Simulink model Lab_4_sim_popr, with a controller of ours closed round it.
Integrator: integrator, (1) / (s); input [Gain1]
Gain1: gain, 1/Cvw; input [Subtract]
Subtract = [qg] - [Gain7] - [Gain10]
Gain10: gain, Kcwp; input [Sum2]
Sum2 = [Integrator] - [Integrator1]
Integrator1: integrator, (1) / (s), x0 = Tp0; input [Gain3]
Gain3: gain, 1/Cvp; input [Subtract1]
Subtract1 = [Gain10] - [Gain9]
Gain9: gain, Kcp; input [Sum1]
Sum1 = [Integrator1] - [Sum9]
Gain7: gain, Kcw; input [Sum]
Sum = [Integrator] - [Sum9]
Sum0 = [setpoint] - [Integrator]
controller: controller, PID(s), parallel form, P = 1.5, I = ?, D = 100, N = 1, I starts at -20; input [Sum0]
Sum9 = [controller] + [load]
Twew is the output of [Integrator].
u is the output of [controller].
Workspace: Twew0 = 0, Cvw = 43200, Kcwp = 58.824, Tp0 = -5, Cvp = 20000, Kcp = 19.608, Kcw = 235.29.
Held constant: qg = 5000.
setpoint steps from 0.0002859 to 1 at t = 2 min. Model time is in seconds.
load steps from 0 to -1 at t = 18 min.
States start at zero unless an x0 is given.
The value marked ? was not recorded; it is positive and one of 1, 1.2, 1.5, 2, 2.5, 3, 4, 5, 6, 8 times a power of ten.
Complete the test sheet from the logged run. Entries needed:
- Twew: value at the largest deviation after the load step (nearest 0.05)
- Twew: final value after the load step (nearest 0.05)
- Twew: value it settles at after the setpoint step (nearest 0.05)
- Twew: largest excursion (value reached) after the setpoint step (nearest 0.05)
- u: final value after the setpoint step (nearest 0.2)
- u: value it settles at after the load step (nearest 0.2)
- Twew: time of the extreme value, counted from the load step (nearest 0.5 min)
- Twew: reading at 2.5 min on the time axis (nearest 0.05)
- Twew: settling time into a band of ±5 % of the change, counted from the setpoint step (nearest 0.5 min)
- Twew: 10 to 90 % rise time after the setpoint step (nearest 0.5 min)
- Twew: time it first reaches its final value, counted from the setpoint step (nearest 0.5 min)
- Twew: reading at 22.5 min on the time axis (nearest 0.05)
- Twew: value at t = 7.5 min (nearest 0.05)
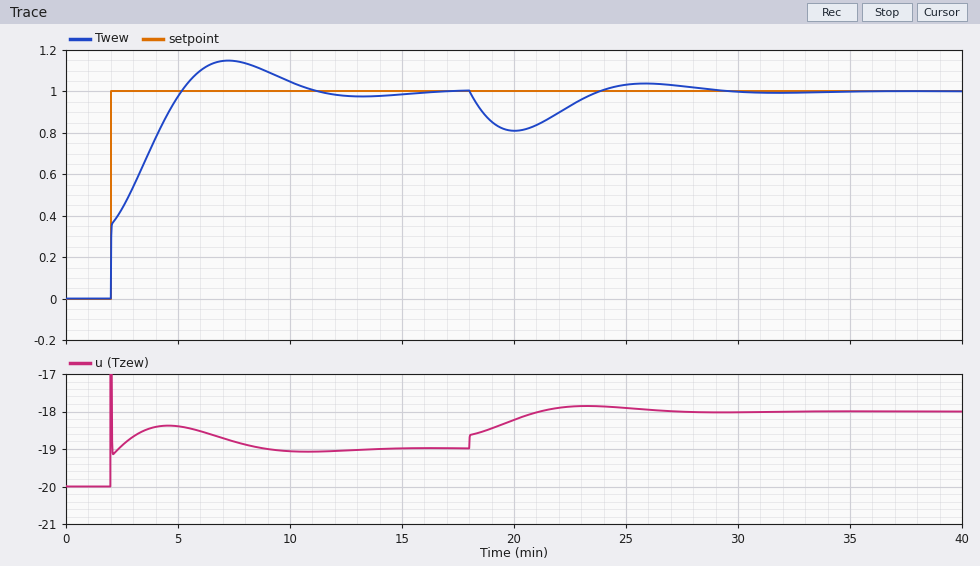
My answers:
0.80
1.00
1.00
1.15
-19.0
-18.0
2.0 min
0.45
8.0 min
2.5 min
3.0 min
0.95
1.15
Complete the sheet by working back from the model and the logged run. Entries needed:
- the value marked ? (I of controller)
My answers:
0.03
